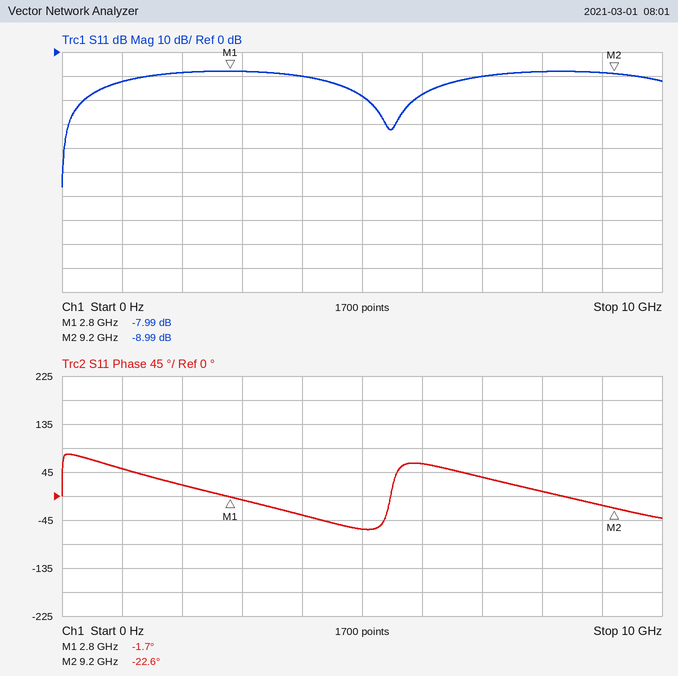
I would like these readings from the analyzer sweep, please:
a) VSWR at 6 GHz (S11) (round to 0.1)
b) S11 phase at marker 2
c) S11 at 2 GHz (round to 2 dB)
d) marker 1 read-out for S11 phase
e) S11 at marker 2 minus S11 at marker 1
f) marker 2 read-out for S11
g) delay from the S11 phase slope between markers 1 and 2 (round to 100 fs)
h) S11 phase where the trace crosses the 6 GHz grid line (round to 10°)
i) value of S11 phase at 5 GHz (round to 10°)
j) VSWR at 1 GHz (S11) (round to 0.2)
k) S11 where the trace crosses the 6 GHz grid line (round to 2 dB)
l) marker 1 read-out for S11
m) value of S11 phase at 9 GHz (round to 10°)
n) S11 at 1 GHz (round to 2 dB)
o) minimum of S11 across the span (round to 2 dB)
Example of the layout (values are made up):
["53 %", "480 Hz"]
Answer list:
["1.3", "-22.6°", "-8 dB", "-1.7°", "-1.00 dB", "-8.99 dB", "9.1 ps", "60°", "-60°", "1.6", "-18 dB", "-7.99 dB", "-20°", "-12 dB", "-56 dB"]
